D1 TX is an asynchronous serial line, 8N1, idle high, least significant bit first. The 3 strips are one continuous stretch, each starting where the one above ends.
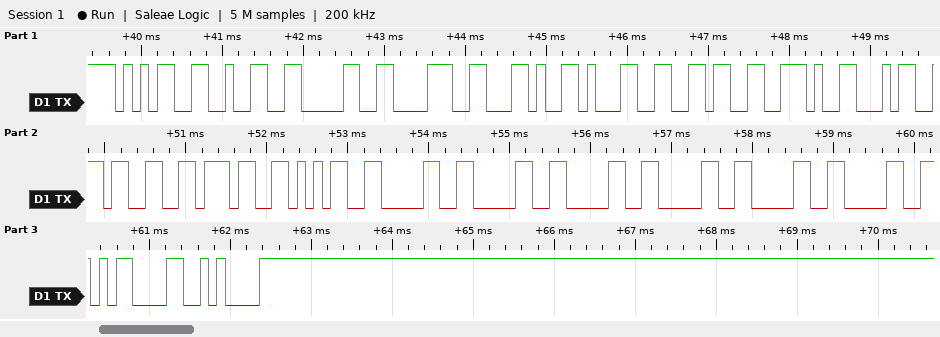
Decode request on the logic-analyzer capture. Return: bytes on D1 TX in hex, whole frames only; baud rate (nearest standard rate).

35 32 30 38 2C 31 36 2E 34 33 37 35 30 30 30 30 30 30 0D 0A
9600 baud
